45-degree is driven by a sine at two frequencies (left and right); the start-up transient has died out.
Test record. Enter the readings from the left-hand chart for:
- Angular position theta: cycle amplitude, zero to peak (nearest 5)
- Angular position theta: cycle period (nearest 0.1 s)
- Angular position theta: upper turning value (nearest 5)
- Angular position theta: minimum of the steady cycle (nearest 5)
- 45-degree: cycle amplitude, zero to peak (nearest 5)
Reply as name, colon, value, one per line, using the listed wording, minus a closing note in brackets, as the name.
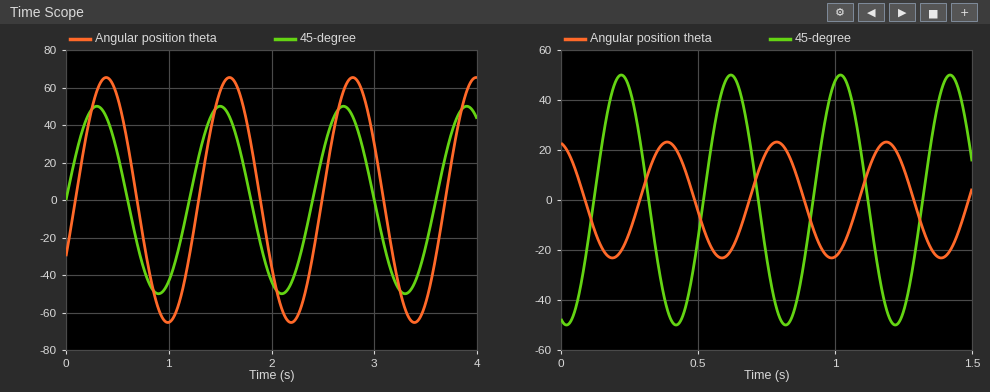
Angular position theta: cycle amplitude, zero to peak: 65
Angular position theta: cycle period: 1.2 s
Angular position theta: upper turning value: 65
Angular position theta: minimum of the steady cycle: -65
45-degree: cycle amplitude, zero to peak: 50
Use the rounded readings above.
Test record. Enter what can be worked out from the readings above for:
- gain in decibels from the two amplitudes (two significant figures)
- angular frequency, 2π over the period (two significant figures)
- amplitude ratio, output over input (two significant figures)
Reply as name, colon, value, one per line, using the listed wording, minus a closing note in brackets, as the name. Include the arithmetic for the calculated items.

gain in decibels from the two amplitudes: 20 log10(65 / 50) = 2.3 dB
angular frequency, 2π over the period: 2π / 1.2 = 5.2 rad/s
amplitude ratio, output over input: 65 / 50 = 1.3
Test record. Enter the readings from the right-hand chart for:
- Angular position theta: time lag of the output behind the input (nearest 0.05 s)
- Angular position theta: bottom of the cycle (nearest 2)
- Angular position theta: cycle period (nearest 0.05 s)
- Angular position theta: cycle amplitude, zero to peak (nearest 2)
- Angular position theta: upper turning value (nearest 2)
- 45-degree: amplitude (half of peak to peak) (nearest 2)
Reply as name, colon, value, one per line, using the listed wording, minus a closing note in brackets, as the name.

Angular position theta: time lag of the output behind the input: 0.15 s
Angular position theta: bottom of the cycle: -24
Angular position theta: cycle period: 0.40 s
Angular position theta: cycle amplitude, zero to peak: 24
Angular position theta: upper turning value: 24
45-degree: amplitude (half of peak to peak): 50
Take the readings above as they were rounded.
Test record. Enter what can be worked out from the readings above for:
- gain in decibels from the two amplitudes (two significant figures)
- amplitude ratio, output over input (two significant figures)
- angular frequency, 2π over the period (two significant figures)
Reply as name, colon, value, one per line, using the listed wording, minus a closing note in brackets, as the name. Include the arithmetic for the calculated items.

gain in decibels from the two amplitudes: 20 log10(24 / 50) = -6.4 dB
amplitude ratio, output over input: 24 / 50 = 0.48
angular frequency, 2π over the period: 2π / 0.4 = 16 rad/s
